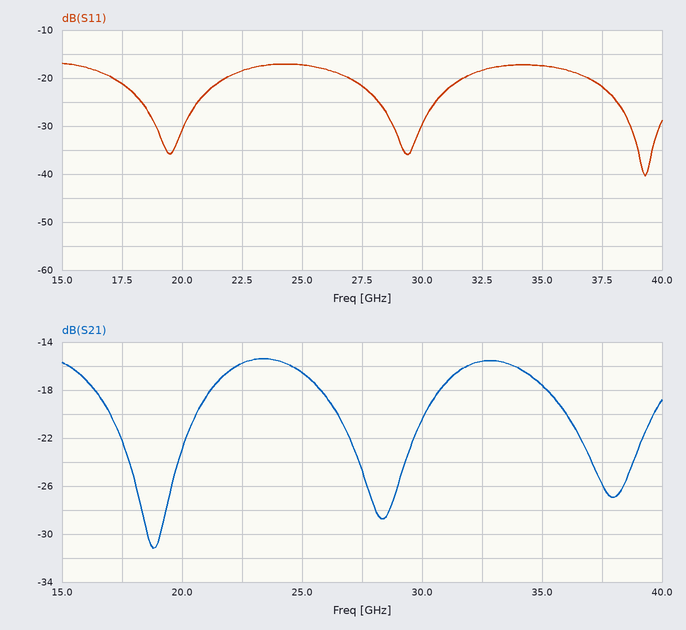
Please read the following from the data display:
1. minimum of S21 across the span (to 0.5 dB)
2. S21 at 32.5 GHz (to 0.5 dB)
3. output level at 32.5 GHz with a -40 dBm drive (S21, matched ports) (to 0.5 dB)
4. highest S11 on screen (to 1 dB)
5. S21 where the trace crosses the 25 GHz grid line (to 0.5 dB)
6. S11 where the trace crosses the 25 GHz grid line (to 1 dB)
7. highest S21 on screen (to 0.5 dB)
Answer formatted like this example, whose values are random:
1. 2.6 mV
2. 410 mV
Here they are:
1. -31.0 dB
2. -15.5 dB
3. -55.5 dBm
4. -17 dB
5. -16.5 dB
6. -17 dB
7. -15.5 dB
